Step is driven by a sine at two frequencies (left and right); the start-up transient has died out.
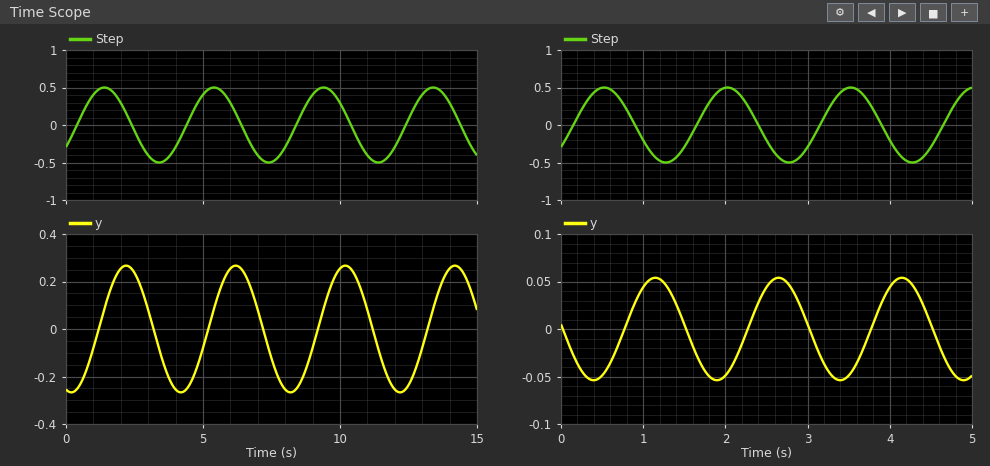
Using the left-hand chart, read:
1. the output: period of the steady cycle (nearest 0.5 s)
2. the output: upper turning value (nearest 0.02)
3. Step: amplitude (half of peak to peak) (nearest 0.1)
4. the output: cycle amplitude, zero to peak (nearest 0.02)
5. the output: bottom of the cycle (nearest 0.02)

4.0 s
0.26
0.5
0.26
-0.26
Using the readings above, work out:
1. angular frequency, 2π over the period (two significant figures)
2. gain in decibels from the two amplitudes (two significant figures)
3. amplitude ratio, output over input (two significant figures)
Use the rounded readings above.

1.6 rad/s
-5.7 dB
0.52
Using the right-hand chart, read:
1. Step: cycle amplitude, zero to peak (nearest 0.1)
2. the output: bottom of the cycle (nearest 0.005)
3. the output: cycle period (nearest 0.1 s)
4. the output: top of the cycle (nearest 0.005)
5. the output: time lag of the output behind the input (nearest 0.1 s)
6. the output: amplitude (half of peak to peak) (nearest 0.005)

0.5
-0.055
1.5 s
0.055
0.6 s
0.055
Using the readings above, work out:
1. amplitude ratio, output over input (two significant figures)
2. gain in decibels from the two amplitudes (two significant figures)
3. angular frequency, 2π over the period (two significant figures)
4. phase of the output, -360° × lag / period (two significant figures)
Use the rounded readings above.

0.11
-19 dB
4.2 rad/s
-140°
